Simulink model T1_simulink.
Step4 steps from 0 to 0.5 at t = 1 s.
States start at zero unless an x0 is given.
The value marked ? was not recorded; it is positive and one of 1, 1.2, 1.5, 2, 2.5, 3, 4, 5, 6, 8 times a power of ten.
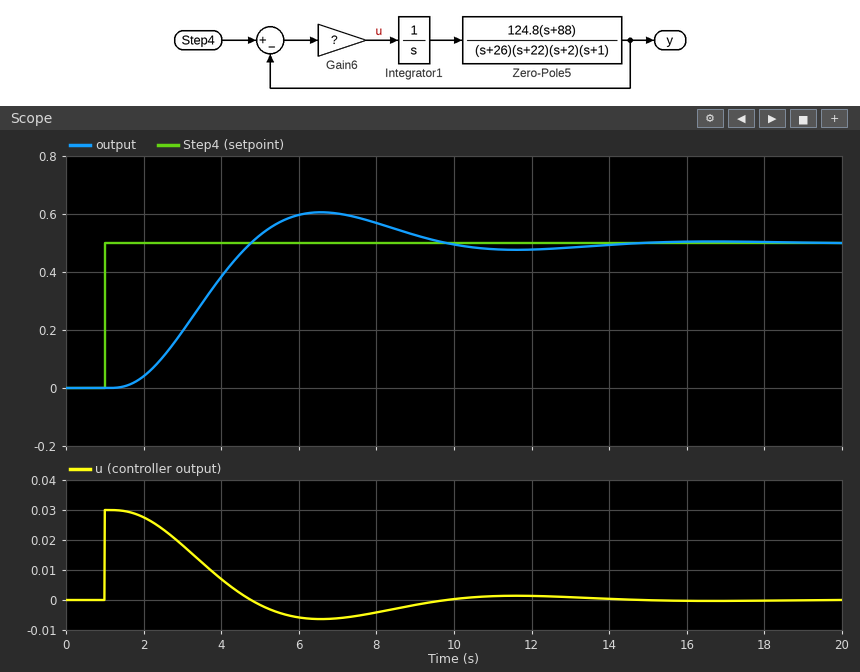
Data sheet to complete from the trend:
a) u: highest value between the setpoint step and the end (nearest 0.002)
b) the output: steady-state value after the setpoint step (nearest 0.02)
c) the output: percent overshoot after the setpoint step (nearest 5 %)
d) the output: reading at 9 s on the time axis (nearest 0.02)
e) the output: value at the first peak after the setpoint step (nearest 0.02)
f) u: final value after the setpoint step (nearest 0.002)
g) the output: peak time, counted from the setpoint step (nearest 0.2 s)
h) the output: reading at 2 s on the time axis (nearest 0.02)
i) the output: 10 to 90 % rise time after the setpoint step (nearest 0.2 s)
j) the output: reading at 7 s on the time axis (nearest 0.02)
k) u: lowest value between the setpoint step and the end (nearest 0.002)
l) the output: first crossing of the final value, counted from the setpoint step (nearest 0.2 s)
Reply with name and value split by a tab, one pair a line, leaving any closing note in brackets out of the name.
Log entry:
u: highest value between the setpoint step and the end	0.030
the output: steady-state value after the setpoint step	0.50
the output: percent overshoot after the setpoint step	20 %
the output: reading at 9 s on the time axis	0.52
the output: value at the first peak after the setpoint step	0.60
u: final value after the setpoint step	0.000
the output: peak time, counted from the setpoint step	5.6 s
the output: reading at 2 s on the time axis	0.04
the output: 10 to 90 % rise time after the setpoint step	2.4 s
the output: reading at 7 s on the time axis	0.60
u: lowest value between the setpoint step and the end	-0.006
the output: first crossing of the final value, counted from the setpoint step	3.8 s
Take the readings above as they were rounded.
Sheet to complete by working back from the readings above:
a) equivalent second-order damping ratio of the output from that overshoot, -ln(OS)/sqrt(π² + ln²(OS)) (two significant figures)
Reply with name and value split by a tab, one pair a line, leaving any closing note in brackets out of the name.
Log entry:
equivalent second-order damping ratio of the output from that overshoot, -ln(OS)/sqrt(π² + ln²(OS))	0.46
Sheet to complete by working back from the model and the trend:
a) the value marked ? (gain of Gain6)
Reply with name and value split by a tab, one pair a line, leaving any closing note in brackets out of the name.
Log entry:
the value marked ?	0.06
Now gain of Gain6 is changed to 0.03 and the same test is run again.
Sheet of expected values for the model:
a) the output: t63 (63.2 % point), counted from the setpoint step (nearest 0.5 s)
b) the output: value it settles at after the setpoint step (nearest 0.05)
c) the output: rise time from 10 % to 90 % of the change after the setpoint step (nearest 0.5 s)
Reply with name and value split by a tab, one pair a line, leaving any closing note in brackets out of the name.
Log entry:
the output: t63 (63.2 % point), counted from the setpoint step	4.0 s
the output: value it settles at after the setpoint step	0.50
the output: rise time from 10 % to 90 % of the change after the setpoint step	4.5 s
